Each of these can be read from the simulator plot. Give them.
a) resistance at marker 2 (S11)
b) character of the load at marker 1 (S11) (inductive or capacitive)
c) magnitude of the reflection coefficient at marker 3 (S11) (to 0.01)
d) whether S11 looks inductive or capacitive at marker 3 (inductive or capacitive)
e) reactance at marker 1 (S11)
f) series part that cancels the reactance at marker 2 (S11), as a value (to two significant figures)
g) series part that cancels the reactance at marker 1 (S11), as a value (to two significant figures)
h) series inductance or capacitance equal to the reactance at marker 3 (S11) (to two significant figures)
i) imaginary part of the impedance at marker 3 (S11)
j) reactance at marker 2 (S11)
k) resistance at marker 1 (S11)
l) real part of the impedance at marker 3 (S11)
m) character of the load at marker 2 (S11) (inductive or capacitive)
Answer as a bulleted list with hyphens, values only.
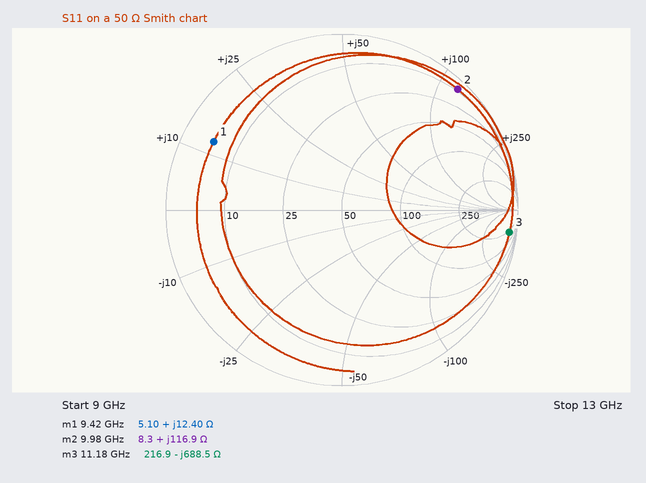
- 8.3 Ω
- inductive
- 0.96
- capacitive
- +12.40 Ω
- 140 fF
- 1.4 pF
- 21 fF
- -688.5 Ω
- +116.9 Ω
- 5.10 Ω
- 216.9 Ω
- inductive
